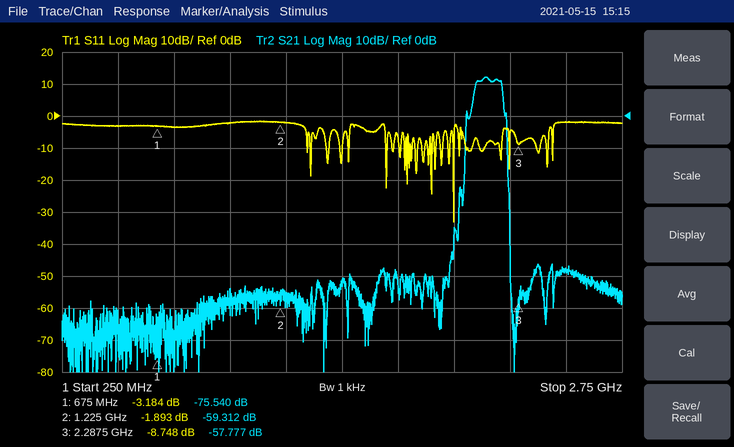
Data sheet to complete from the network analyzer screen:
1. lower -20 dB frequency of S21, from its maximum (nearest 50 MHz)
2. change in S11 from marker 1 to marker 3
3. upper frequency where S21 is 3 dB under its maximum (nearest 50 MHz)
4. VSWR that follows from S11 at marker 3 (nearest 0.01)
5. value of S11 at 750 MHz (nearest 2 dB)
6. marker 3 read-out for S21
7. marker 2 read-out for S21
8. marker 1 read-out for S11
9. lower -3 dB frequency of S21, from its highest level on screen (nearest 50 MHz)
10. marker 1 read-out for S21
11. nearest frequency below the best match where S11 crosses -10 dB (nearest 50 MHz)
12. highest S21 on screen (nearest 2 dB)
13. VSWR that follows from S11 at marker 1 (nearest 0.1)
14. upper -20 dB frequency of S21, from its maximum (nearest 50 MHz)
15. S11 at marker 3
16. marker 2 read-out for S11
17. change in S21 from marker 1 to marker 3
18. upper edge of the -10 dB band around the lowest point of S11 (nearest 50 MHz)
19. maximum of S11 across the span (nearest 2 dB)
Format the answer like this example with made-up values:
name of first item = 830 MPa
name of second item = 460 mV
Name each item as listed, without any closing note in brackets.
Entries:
lower -20 dB frequency of S21, from its maximum = 2.05 GHz
change in S11 from marker 1 to marker 3 = -5.564 dB
upper frequency where S21 is 3 dB under its maximum = 2.20 GHz
VSWR that follows from S11 at marker 3 = 2.15
value of S11 at 750 MHz = -4 dB
marker 3 read-out for S21 = -57.777 dB
marker 2 read-out for S21 = -59.312 dB
marker 1 read-out for S11 = -3.184 dB
lower -3 dB frequency of S21, from its highest level on screen = 2.10 GHz
marker 1 read-out for S21 = -75.540 dB
nearest frequency below the best match where S11 crosses -10 dB = 2.00 GHz
highest S21 on screen = 12 dB
VSWR that follows from S11 at marker 1 = 5.5
upper -20 dB frequency of S21, from its maximum = 2.25 GHz
S11 at marker 3 = -8.748 dB
marker 2 read-out for S11 = -1.893 dB
change in S21 from marker 1 to marker 3 = 17.763 dB
upper edge of the -10 dB band around the lowest point of S11 = 2.00 GHz
maximum of S11 across the span = -2 dB
